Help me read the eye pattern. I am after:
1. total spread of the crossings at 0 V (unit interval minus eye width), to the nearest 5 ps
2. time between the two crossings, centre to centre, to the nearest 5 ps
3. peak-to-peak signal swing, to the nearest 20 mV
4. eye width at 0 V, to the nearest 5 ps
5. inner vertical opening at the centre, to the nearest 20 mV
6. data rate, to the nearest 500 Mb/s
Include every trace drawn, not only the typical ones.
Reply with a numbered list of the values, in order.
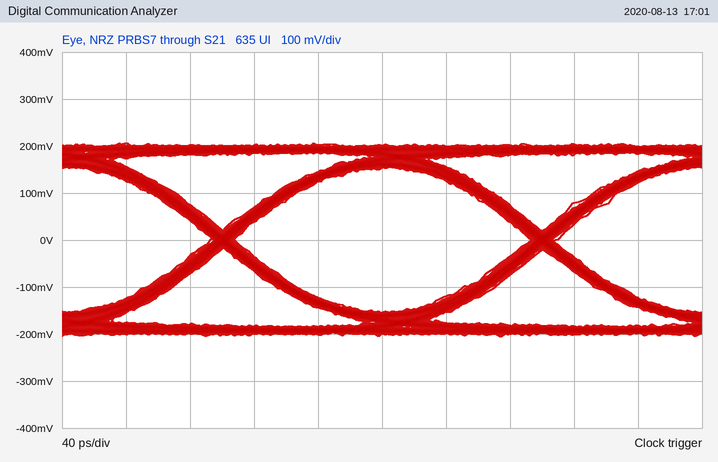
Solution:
1. 15 ps
2. 200 ps
3. 420 mV
4. 185 ps
5. 300 mV
6. 5.0 Gb/s
